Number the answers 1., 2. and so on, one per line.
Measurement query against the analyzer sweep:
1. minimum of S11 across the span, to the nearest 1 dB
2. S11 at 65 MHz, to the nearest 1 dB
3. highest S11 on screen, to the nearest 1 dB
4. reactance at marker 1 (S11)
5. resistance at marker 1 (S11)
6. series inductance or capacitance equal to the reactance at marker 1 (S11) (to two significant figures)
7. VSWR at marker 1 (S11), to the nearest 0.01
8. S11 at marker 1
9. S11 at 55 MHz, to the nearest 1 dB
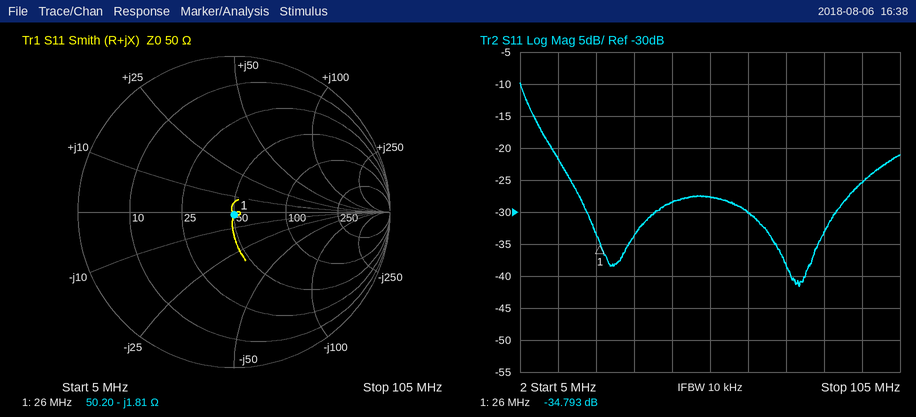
1. -42 dB
2. -30 dB
3. -10 dB
4. -1.81 Ω
5. 50.20 Ω
6. 3.4 nF
7. 1.04
8. -34.793 dB
9. -28 dB
